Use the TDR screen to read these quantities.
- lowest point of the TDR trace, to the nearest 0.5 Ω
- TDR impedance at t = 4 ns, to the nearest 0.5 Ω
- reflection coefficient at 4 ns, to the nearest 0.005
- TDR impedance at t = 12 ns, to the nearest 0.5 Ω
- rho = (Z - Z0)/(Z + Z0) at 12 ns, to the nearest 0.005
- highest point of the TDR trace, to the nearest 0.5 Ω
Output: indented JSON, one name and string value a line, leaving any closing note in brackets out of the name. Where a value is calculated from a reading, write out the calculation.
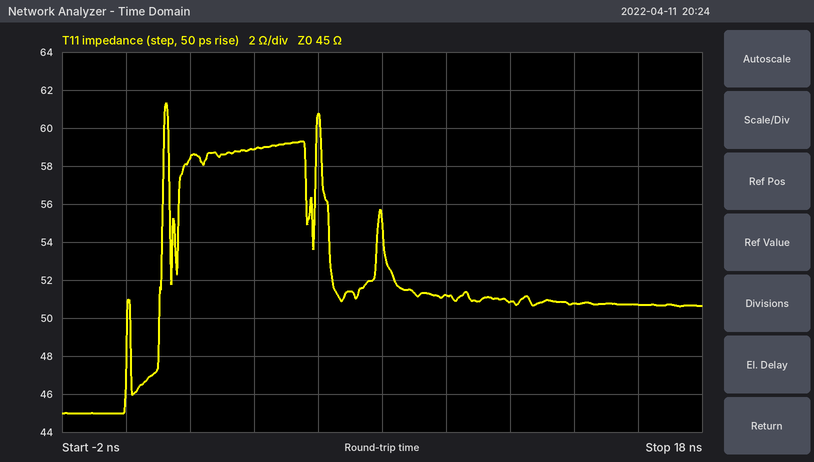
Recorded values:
{
  "lowest point of the TDR trace, to the nearest 0.5 Ω": "45.0 Ω",
  "TDR impedance at t = 4 ns, to the nearest 0.5 Ω": "59.0 Ω",
  "reflection coefficient at 4 ns, to the nearest 0.005": "(59 − 45)/(59 + 45) ≈ +0.135",
  "TDR impedance at t = 12 ns, to the nearest 0.5 Ω": "51.0 Ω",
  "rho = (Z - Z0)/(Z + Z0) at 12 ns, to the nearest 0.005": "(51 − 45)/(51 + 45) ≈ +0.0625, so +0.060 to the nearest 0.005",
  "highest point of the TDR trace, to the nearest 0.5 Ω": "61.5 Ω"
}
